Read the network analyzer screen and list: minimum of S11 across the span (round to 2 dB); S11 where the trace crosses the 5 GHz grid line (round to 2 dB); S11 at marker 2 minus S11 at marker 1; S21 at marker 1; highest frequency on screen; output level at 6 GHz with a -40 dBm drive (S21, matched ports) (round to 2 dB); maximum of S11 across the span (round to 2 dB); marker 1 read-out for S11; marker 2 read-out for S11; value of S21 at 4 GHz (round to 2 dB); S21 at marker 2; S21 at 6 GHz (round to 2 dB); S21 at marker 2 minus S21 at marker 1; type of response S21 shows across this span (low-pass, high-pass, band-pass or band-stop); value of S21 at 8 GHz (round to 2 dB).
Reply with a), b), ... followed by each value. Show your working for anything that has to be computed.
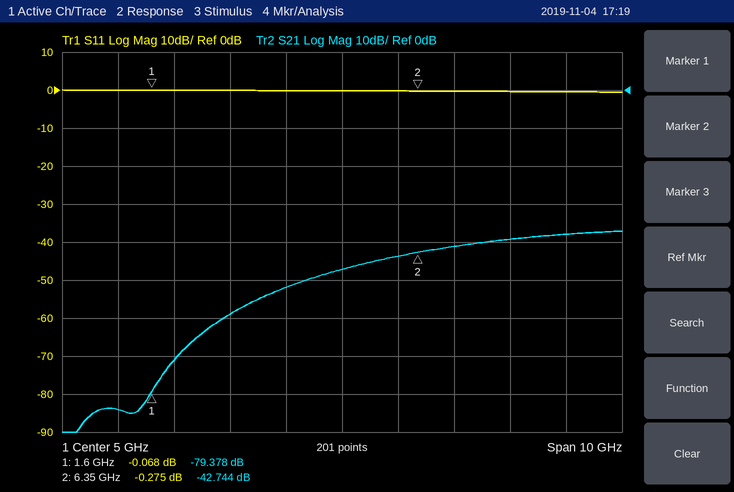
a) 0 dB
b) 0 dB
c) -0.275 − (-0.068) = -0.207 dB
d) -79.378 dB
e) 10 GHz
f) -40 dBm + (-44 dB) = -84 dBm
g) 0 dB
h) -0.068 dB
i) -0.275 dB
j) -52 dB
k) -42.744 dB
l) -44 dB
m) -42.744 − (-79.378) = 36.634 dB
n) high-pass
o) -40 dB
